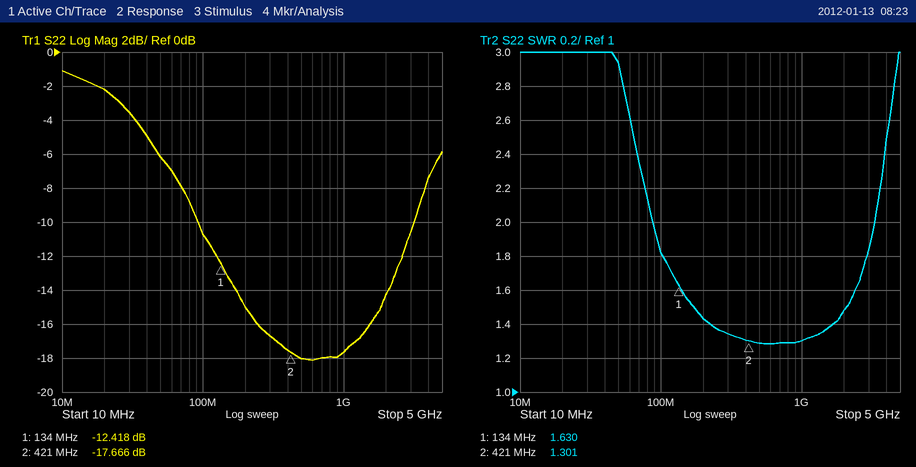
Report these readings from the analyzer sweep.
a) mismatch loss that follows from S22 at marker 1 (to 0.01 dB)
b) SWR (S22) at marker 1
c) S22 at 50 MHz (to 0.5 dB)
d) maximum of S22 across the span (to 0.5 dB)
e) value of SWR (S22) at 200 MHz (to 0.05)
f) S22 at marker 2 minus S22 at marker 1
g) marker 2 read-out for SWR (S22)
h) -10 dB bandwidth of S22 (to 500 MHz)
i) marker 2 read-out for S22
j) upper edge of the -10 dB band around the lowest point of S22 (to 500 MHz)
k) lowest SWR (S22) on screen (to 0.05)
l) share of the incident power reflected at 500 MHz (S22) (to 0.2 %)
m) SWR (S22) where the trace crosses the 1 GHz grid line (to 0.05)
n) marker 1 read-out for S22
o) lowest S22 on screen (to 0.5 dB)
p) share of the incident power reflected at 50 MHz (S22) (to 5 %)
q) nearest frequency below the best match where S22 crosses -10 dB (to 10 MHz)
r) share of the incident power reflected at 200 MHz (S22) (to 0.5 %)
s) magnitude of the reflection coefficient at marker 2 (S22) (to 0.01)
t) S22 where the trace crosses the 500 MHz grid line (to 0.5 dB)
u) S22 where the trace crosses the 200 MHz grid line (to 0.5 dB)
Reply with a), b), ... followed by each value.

a) 0.26 dB
b) 1.630
c) -6.0 dB
d) -1.0 dB
e) 1.45
f) -5.248 dB
g) 1.301
h) 3.0 GHz
i) -17.666 dB
j) 3.0 GHz
k) 1.30
l) 1.6 %
m) 1.30
n) -12.418 dB
o) -18.0 dB
p) 25 %
q) 90 MHz
r) 3.0 %
s) 0.13
t) -18.0 dB
u) -15.0 dB
